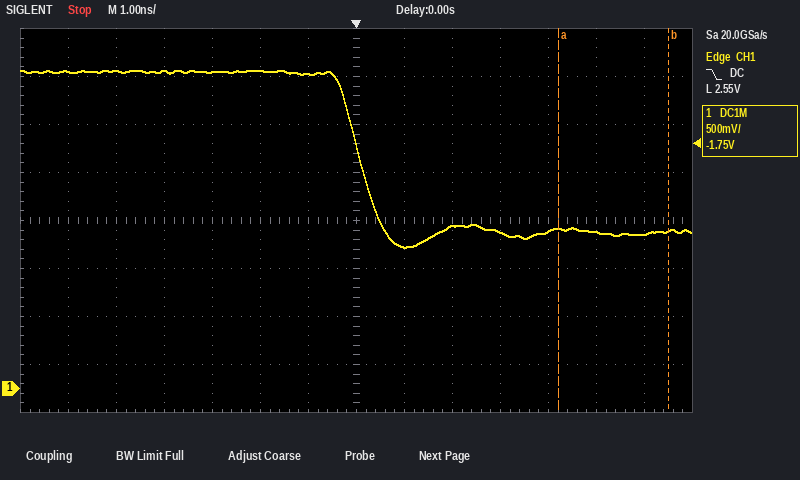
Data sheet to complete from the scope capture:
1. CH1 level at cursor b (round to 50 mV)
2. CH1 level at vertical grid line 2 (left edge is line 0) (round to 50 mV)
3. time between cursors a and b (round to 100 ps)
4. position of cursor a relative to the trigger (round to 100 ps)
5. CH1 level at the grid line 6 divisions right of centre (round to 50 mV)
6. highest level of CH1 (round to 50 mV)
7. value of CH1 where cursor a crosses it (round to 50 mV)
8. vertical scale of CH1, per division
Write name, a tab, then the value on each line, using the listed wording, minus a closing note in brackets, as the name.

CH1 level at cursor b	1.65 V
CH1 level at vertical grid line 2 (left edge is line 0)	3.30 V
time between cursors a and b	2.3 ns
position of cursor a relative to the trigger	+4.2 ns
CH1 level at the grid line 6 divisions right of centre	1.60 V
highest level of CH1	3.30 V
value of CH1 where cursor a crosses it	1.65 V
vertical scale of CH1, per division	500 mV
